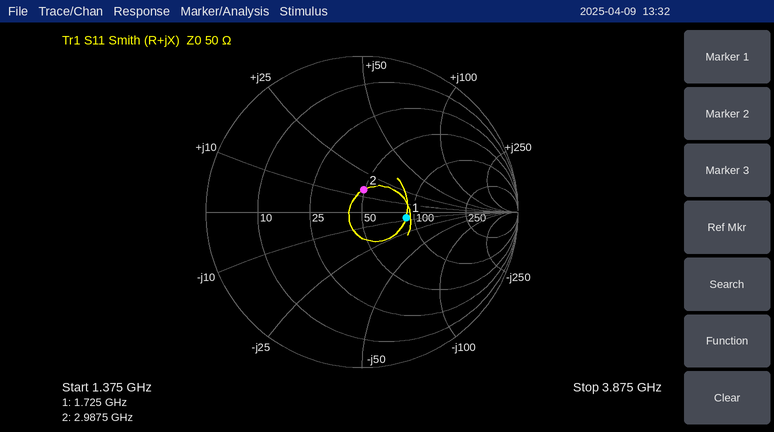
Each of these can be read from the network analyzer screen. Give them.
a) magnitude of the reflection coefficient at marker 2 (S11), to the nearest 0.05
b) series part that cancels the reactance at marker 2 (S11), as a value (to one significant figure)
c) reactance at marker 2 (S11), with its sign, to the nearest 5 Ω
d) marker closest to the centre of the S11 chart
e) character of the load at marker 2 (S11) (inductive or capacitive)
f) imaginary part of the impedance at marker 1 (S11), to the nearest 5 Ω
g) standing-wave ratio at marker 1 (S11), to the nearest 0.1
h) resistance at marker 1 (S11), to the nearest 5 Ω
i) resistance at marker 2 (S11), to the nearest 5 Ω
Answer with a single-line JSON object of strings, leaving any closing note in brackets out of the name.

{"magnitude of the reflection coefficient at marker 2 (S11), to the nearest 0.05": "0.15", "series part that cancels the reactance at marker 2 (S11), as a value": "4 pF", "reactance at marker 2 (S11), with its sign, to the nearest 5 Ω": "+15 Ω", "marker closest to the centre of the S11 chart": "marker 2", "character of the load at marker 2 (S11)": "inductive", "imaginary part of the impedance at marker 1 (S11), to the nearest 5 Ω": "-5 Ω", "standing-wave ratio at marker 1 (S11), to the nearest 0.1": "1.8", "resistance at marker 1 (S11), to the nearest 5 Ω": "90 Ω", "resistance at marker 2 (S11), to the nearest 5 Ω": "50 Ω"}
